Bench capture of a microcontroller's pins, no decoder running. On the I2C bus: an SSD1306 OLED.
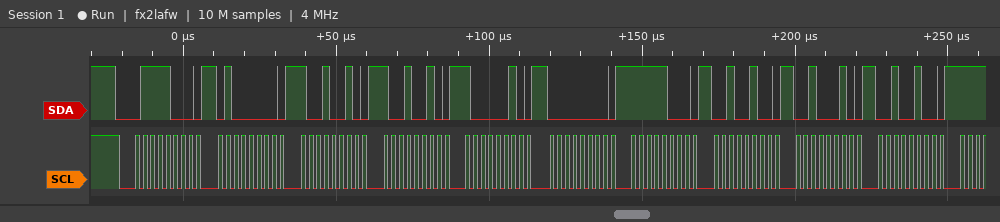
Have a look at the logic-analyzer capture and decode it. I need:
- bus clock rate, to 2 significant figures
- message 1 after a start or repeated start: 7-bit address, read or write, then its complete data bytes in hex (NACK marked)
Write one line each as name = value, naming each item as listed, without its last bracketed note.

bus clock rate, to 2 significant figures = 400 kHz
message 1 after a start or repeated start: 7-bit address, read or write, then its complete data bytes in hex = 0x3C write: 40 92 92 82 00 F8 24 22 24
